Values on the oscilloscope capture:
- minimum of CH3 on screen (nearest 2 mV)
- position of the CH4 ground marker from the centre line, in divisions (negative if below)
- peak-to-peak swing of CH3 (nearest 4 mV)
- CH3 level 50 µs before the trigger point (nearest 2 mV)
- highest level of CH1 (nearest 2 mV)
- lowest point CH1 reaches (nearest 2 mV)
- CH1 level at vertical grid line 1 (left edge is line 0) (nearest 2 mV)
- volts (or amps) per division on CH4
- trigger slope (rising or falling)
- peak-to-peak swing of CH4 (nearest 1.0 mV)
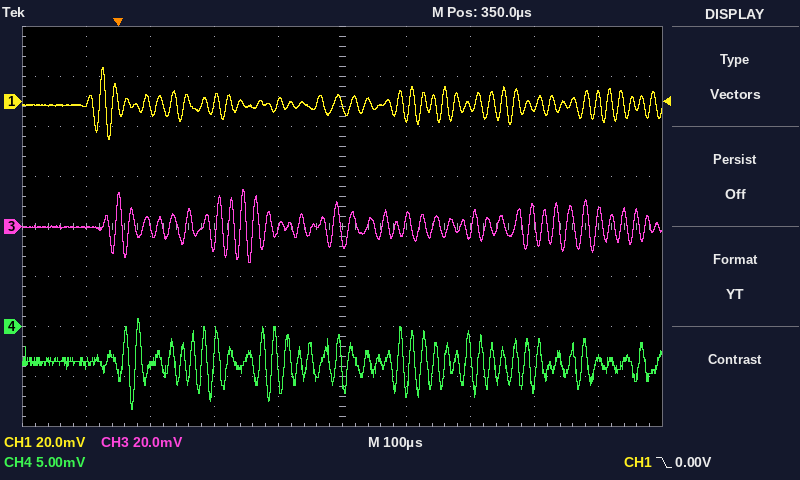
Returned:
-14 mV
-2.0 div
28 mV
0 mV
14 mV
-16 mV
0 mV
5 mV
falling
9.0 mV
